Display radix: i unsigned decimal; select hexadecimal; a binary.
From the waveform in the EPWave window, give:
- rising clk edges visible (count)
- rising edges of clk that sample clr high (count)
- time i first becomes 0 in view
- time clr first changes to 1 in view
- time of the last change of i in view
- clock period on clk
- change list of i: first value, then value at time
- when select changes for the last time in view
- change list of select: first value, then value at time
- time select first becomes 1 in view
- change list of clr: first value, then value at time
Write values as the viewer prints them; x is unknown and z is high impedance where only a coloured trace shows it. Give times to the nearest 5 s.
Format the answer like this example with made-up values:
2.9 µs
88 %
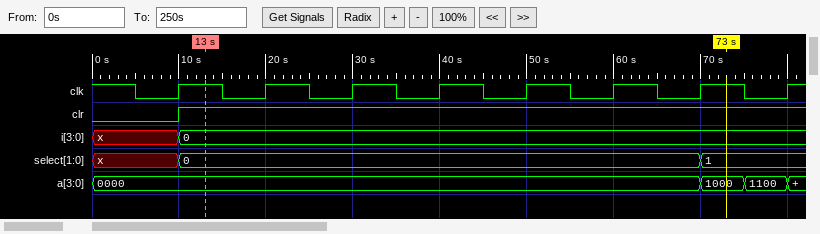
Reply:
8
7
10 s
10 s
10 s
10 s
x, 0 at 10 s
70 s
x, 0 at 10 s, 1 at 70 s
70 s
0, 1 at 10 s
